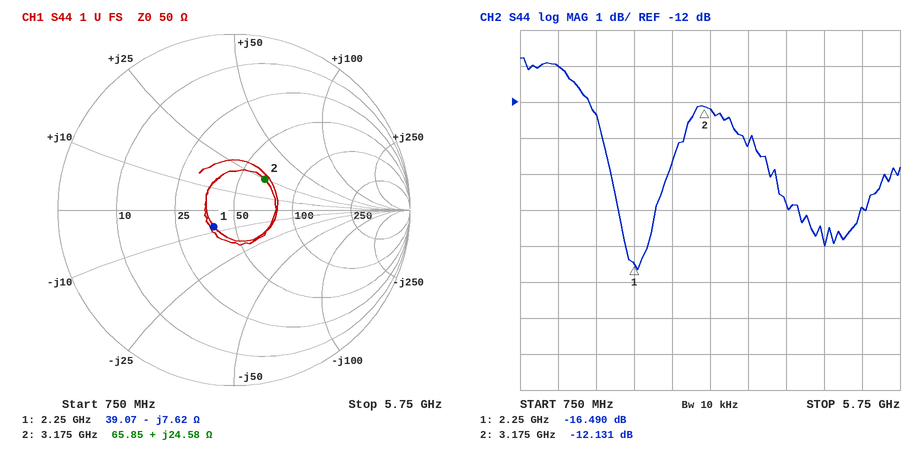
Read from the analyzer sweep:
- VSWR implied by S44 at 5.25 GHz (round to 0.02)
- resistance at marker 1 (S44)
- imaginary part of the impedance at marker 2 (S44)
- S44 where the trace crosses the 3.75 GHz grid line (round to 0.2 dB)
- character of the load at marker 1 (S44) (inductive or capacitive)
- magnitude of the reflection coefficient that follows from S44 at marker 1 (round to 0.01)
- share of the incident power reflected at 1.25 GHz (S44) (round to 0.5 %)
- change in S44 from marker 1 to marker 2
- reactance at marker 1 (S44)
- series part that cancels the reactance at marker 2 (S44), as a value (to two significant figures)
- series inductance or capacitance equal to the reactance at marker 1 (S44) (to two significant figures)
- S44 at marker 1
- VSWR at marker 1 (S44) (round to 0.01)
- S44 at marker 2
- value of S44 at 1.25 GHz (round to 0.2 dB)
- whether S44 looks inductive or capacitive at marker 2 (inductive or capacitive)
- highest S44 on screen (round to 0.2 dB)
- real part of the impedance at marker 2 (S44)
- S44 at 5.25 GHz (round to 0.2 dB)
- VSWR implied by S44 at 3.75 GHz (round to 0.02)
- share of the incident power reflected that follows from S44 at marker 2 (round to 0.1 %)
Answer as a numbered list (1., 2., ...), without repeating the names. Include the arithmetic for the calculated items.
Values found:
1. |Γ| = 10^(-15/20) = 0.1778; VSWR = (1 + 0.1778)/(1 − 0.1778) ≈ 1.43, so 1.44 to the nearest 0.02
2. 39.07 Ω
3. +24.58 Ω
4. -13.2 dB
5. capacitive
6. 10^(-16.49/20) ≈ 0.15
7. 10^(-11/10) ≈ 7.94 %, so 8.0 % to the nearest 0.5 %
8. -12.131 − (-16.49) = 4.359 dB
9. -7.62 Ω
10. C = 1/(2π × 3.175 GHz × 24.58 Ω) ≈ 2.0 pF
11. C = 1/(2π × 2.25 GHz × 7.62 Ω) ≈ 9.3 pF
12. -16.490 dB
13. 1.35
14. -12.131 dB
15. -11.0 dB
16. inductive
17. -10.8 dB
18. 65.85 Ω
19. -15.0 dB
20. |Γ| = 10^(-13.2/20) = 0.2188; VSWR = (1 + 0.2188)/(1 − 0.2188) ≈ 1.56
21. 10^(-12.131/10) ≈ 6.1 %
